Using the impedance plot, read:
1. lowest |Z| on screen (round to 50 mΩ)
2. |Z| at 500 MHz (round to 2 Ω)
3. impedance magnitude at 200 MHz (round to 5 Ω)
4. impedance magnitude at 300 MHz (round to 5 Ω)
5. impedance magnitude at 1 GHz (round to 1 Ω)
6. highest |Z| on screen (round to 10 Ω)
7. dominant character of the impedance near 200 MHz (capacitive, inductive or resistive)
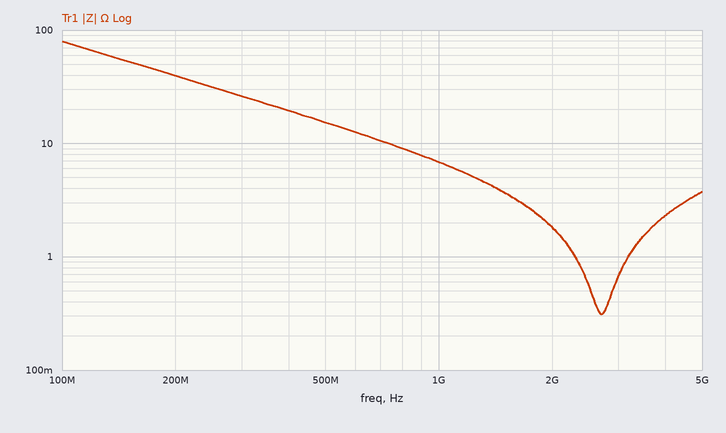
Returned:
300 mΩ
16 Ω
40 Ω
25 Ω
7 Ω
80 Ω
capacitive
